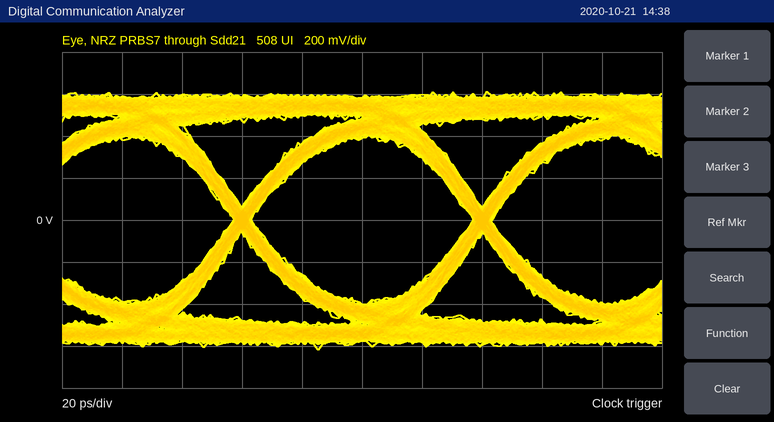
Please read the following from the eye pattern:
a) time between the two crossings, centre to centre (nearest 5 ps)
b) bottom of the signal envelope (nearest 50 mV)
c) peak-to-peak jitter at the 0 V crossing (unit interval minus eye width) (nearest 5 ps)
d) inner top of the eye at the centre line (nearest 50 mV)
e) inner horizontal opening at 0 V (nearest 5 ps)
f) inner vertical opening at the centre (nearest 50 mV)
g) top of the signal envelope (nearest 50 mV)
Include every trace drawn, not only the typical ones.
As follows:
80 ps
-600 mV
5 ps
400 mV
75 ps
800 mV
600 mV
